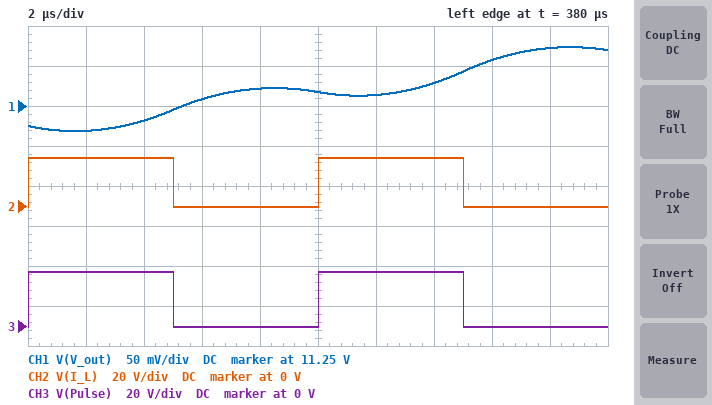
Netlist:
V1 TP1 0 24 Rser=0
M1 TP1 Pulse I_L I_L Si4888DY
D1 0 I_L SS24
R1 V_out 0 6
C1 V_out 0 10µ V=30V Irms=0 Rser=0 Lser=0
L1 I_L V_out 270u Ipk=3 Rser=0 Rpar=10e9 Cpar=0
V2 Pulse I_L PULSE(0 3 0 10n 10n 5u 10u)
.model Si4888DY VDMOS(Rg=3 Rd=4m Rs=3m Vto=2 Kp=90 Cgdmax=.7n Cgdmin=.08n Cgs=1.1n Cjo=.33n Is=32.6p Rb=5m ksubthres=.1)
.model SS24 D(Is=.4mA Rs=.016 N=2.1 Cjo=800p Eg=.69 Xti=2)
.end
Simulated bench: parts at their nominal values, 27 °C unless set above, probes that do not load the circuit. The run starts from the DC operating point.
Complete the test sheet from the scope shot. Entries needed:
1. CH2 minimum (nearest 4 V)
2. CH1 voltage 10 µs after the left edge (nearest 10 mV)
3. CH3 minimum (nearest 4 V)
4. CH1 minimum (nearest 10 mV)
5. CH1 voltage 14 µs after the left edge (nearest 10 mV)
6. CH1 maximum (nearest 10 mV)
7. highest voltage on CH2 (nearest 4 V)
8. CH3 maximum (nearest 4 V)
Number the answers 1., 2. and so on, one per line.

1. 0 V
2. 11.27 V
3. 0 V
4. 11.22 V
5. 11.28 V
6. 11.32 V
7. 24 V
8. 28 V
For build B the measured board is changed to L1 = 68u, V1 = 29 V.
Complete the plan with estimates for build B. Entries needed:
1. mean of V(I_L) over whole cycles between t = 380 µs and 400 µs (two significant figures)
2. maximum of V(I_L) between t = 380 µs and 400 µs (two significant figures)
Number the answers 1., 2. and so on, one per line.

1. 14 V
2. 29 V
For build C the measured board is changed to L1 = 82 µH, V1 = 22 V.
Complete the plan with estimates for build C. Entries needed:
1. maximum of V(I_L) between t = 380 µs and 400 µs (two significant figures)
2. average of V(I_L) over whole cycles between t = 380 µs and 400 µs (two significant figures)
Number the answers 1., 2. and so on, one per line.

1. 22 V
2. 11 V
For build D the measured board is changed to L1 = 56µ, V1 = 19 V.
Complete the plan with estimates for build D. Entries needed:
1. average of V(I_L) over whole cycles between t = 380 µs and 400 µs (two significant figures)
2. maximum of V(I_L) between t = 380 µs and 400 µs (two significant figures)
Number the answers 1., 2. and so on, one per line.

1. 9.3 V
2. 19 V
